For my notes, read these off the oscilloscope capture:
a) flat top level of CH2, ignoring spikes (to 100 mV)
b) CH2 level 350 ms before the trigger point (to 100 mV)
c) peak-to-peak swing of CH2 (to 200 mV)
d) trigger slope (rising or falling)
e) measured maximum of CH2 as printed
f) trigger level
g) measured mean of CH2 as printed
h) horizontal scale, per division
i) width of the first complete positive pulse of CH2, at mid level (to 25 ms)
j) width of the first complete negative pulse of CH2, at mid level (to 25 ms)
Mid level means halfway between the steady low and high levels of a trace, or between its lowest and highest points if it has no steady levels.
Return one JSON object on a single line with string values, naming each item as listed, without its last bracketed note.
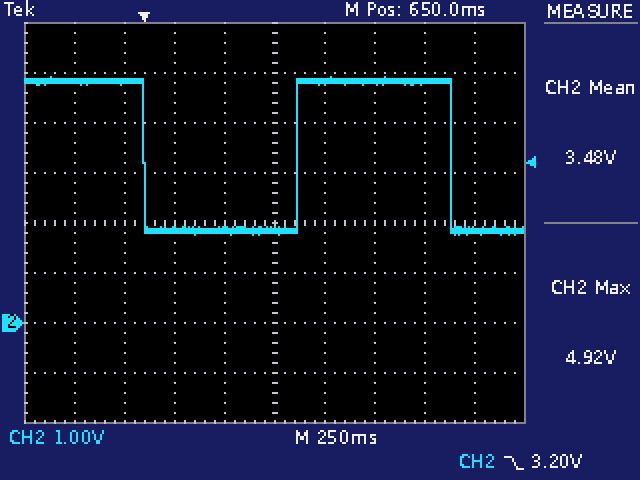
{"flat top level of CH2, ignoring spikes": "4.8 V", "CH2 level 350 ms before the trigger point": "4.8 V", "peak-to-peak swing of CH2": "3.2 V", "trigger slope": "falling", "measured maximum of CH2 as printed": "4.92 V", "trigger level": "3.20 V", "measured mean of CH2 as printed": "3.48 V", "horizontal scale, per division": "250 ms", "width of the first complete positive pulse of CH2, at mid level": "775 ms", "width of the first complete negative pulse of CH2, at mid level": "775 ms"}
